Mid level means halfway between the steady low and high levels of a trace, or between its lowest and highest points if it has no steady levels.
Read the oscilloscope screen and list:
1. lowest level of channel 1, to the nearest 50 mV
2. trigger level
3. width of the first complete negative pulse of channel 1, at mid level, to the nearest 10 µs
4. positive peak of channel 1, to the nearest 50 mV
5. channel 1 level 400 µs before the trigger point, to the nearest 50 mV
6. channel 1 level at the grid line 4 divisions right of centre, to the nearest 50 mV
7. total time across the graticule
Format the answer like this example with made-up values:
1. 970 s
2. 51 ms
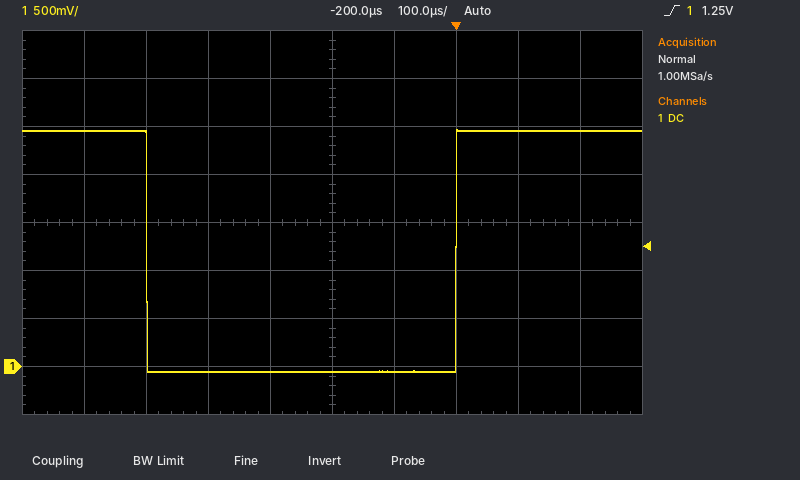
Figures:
1. -50 mV
2. 1.25 V
3. 500 µs
4. 2.45 V
5. -50 mV
6. 2.45 V
7. 1 ms
